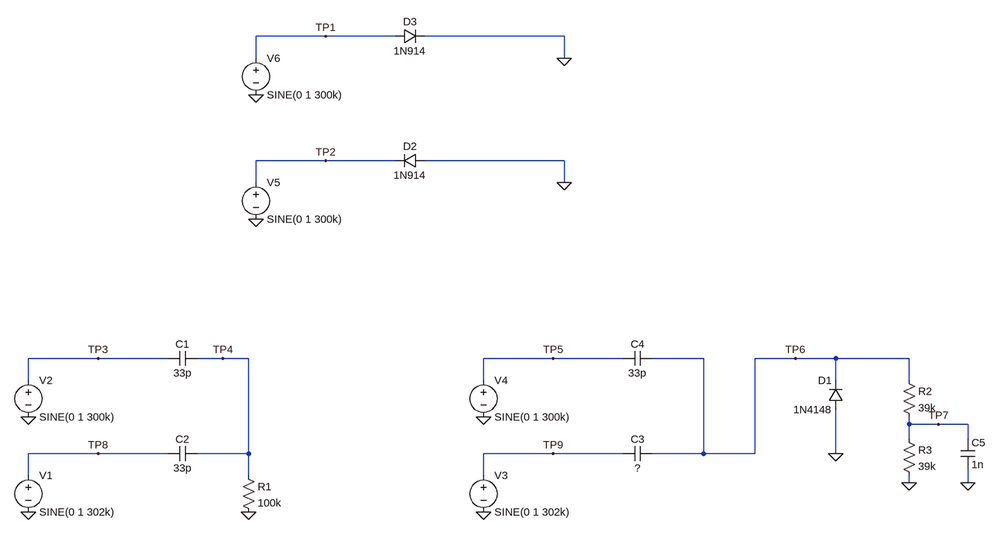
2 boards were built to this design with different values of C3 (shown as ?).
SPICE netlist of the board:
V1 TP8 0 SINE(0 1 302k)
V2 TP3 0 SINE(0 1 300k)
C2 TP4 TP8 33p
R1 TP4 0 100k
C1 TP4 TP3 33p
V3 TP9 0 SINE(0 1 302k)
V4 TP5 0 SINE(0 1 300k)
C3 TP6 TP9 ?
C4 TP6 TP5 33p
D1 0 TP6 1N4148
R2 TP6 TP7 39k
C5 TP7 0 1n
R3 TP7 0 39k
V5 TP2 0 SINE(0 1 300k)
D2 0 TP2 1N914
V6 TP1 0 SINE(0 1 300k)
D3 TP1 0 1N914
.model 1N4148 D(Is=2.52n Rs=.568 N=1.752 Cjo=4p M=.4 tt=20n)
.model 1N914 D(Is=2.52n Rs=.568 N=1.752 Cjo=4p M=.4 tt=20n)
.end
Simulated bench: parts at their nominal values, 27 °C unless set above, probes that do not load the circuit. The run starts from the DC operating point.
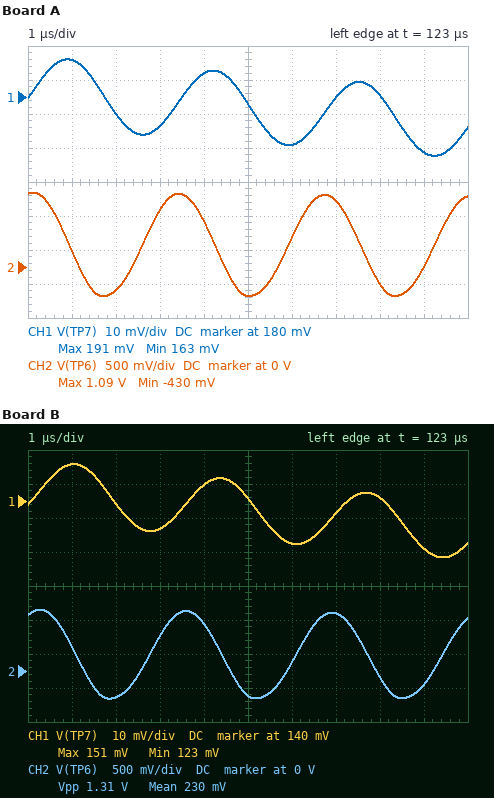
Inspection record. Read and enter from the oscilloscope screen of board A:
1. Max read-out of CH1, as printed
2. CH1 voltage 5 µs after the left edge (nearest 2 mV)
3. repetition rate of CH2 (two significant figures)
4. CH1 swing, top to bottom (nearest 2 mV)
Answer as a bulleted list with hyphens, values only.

- 191 mV
- 178 mV
- 300 kHz
- 28 mV
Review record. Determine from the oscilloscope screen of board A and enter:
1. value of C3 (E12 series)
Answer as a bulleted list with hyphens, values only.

- 100 pF
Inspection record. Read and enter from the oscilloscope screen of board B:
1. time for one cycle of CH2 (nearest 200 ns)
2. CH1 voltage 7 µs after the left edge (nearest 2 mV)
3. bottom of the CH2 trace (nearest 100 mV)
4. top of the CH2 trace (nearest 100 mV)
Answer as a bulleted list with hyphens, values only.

- 3.4 µs
- 136 mV
- -400 mV
- 900 mV
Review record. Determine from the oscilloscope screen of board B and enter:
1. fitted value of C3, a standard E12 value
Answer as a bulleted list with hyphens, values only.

- 39 pF
